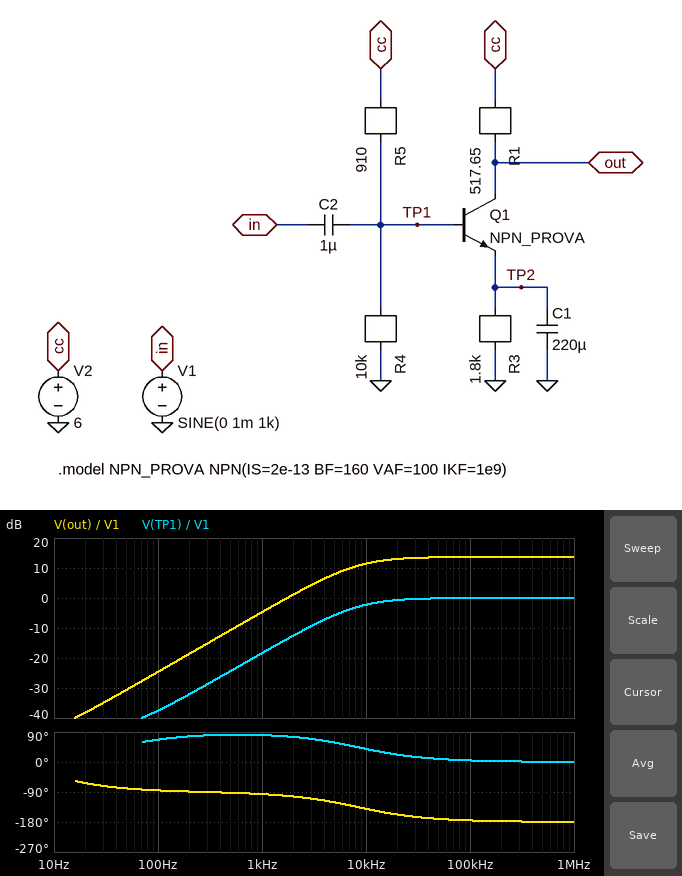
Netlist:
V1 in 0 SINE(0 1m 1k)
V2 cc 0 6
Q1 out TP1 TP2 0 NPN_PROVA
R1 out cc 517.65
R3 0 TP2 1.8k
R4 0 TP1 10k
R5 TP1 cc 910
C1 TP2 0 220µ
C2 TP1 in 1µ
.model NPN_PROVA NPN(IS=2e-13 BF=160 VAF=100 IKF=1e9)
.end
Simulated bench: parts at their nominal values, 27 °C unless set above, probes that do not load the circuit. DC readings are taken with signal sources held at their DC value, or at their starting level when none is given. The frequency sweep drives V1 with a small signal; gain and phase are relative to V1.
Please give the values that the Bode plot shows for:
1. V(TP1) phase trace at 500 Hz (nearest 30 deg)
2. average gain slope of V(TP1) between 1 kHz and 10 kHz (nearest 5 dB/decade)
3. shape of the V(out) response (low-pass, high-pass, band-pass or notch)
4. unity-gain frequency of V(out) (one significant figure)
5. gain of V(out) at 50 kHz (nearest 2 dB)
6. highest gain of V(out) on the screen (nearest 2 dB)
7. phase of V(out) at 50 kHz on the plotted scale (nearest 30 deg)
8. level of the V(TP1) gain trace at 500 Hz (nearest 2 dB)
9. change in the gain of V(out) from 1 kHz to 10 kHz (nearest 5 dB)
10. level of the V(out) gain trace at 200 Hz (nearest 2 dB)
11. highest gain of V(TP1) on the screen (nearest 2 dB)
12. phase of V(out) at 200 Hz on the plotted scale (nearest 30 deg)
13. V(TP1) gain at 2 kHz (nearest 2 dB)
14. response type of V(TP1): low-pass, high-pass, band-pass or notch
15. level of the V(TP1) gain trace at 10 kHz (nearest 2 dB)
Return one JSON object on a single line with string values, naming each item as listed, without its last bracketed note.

{"V(TP1) phase trace at 500 Hz": "90 deg", "average gain slope of V(TP1) between 1 kHz and 10 kHz": "15 dB/decade", "shape of the V(out) response": "high-pass", "unity-gain frequency of V(out)": "2 kHz", "gain of V(out) at 50 kHz": "14 dB", "highest gain of V(out) on the screen": "14 dB", "phase of V(out) at 50 kHz on the plotted scale": "-180 deg", "level of the V(TP1) gain trace at 500 Hz": "-24 dB", "change in the gain of V(out) from 1 kHz to 10 kHz": "15 dB", "level of the V(out) gain trace at 200 Hz": "-18 dB", "highest gain of V(TP1) on the screen": "0 dB", "phase of V(out) at 200 Hz on the plotted scale": "-90 deg", "V(TP1) gain at 2 kHz": "-12 dB", "response type of V(TP1): low-pass, high-pass, band-pass or notch": "high-pass", "level of the V(TP1) gain trace at 10 kHz": "-2 dB"}
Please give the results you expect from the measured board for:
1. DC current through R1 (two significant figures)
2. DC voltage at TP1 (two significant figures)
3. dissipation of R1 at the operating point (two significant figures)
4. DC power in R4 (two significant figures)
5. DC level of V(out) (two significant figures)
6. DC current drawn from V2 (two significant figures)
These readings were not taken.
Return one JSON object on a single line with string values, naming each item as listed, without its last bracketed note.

{"DC current through R1": "2.4 mA", "DC voltage at TP1": "5.3 V", "dissipation of R1 at the operating point": "2.9 mW", "DC power in R4": "2.8 mW", "DC level of V(out)": "4.8 V", "DC current drawn from V2": "3.1 mA"}
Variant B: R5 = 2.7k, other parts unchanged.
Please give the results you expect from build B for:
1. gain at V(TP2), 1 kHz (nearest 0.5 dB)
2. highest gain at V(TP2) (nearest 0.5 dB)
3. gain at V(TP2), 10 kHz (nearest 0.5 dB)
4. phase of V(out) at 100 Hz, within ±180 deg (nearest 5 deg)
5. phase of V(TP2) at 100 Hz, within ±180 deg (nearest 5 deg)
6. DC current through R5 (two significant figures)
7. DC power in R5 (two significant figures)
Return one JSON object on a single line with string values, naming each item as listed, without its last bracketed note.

{"gain at V(TP2), 1 kHz": "-24.0 dB", "highest gain at V(TP2)": "-11.0 dB", "gain at V(TP2), 10 kHz": "-44.0 dB", "phase of V(out) at 100 Hz, within ±180 deg": "-105 deg", "phase of V(TP2) at 100 Hz, within ±180 deg": "-15 deg", "DC current through R5": "480 µA", "DC power in R5": "630 µW"}
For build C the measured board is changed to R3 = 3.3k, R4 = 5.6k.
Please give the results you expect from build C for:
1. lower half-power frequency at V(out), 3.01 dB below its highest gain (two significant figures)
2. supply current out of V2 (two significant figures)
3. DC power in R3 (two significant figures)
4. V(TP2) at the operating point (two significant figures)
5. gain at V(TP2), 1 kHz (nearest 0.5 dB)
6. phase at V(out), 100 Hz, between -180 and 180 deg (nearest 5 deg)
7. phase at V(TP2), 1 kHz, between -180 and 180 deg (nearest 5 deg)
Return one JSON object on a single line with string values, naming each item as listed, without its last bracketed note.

{"lower half-power frequency at V(out), 3.01 dB below its highest gain": "270 Hz", "supply current out of V2": "2.3 mA", "DC power in R3": "6.3 mW", "V(TP2) at the operating point": "4.6 V", "gain at V(TP2), 1 kHz": "-28.5 dB", "phase at V(out), 100 Hz, between -180 and 180 deg": "-95 deg", "phase at V(TP2), 1 kHz, between -180 and 180 deg": "-75 deg"}
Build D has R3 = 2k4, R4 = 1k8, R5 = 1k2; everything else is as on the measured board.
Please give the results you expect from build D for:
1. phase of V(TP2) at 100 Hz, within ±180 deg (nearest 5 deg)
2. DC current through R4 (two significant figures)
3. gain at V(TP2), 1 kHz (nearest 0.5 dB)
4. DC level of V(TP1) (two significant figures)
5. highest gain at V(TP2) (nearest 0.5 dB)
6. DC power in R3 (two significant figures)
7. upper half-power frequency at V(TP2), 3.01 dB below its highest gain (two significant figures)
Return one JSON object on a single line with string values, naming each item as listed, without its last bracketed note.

{"phase of V(TP2) at 100 Hz, within ±180 deg": "-5 deg", "DC current through R4": "2.0 mA", "gain at V(TP2), 1 kHz": "-29.5 dB", "DC level of V(TP1)": "3.6 V", "highest gain at V(TP2)": "-19.0 dB", "DC power in R3": "3.8 mW", "upper half-power frequency at V(TP2), 3.01 dB below its highest gain": "330 Hz"}
